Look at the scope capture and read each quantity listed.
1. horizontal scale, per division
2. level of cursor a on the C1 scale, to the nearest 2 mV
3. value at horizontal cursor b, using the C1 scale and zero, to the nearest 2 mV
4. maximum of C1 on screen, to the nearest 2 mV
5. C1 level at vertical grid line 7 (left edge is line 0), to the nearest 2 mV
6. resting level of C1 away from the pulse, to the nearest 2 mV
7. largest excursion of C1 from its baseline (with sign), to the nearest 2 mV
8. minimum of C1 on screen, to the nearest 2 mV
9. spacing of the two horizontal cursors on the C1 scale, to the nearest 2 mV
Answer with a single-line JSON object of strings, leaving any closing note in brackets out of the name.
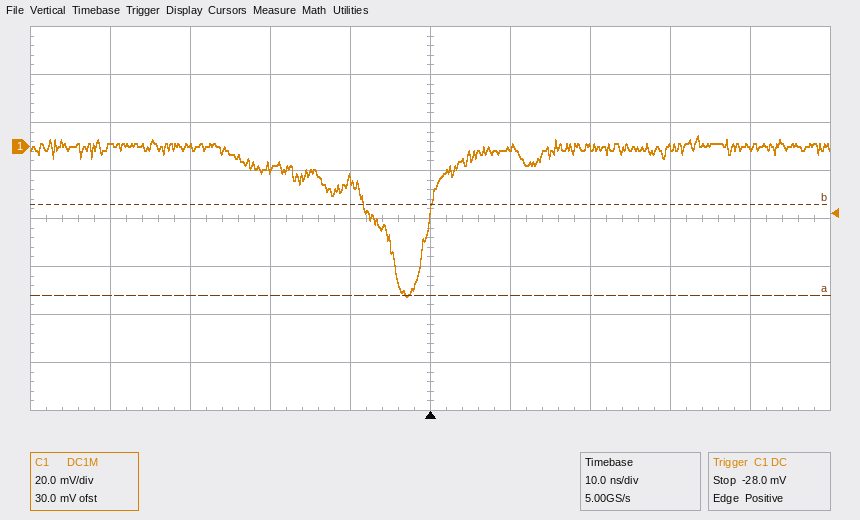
{"horizontal scale, per division": "10 ns", "level of cursor a on the C1 scale, to the nearest 2 mV": "-62 mV", "value at horizontal cursor b, using the C1 scale and zero, to the nearest 2 mV": "-24 mV", "maximum of C1 on screen, to the nearest 2 mV": "4 mV", "C1 level at vertical grid line 7 (left edge is line 0), to the nearest 2 mV": "0 mV", "resting level of C1 away from the pulse, to the nearest 2 mV": "0 mV", "largest excursion of C1 from its baseline (with sign), to the nearest 2 mV": "-62 mV", "minimum of C1 on screen, to the nearest 2 mV": "-62 mV", "spacing of the two horizontal cursors on the C1 scale, to the nearest 2 mV": "38 mV"}
